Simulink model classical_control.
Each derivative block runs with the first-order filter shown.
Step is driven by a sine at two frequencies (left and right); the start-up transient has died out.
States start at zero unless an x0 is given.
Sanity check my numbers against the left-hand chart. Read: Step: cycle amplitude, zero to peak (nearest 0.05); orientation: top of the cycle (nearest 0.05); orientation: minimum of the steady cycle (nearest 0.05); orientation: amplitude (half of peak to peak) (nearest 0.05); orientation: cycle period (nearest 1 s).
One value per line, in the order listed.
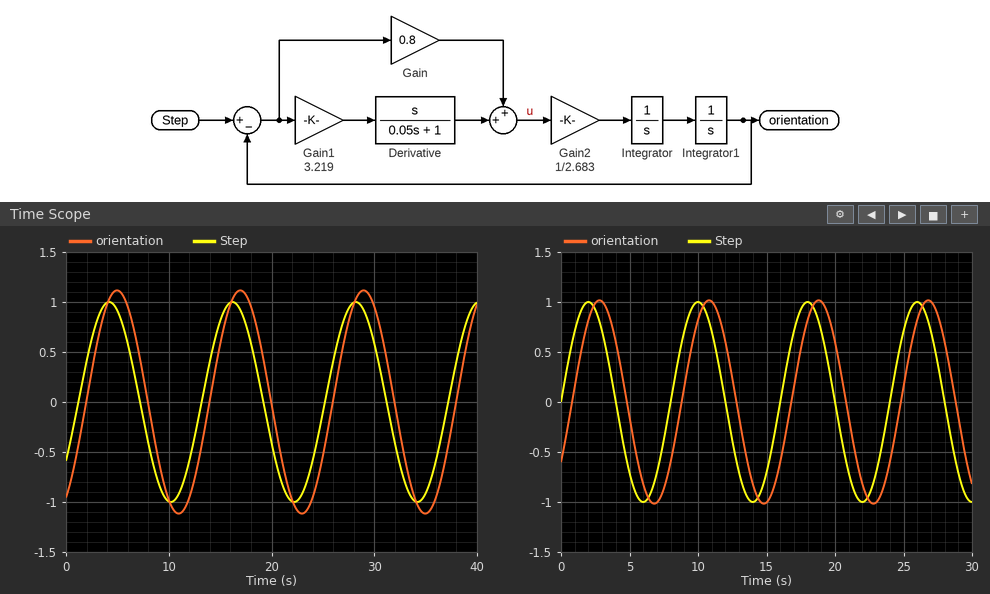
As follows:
1.00
1.10
-1.10
1.10
12 s
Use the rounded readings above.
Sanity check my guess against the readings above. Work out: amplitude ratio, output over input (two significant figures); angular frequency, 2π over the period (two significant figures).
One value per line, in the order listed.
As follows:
1.1
0.52 rad/s
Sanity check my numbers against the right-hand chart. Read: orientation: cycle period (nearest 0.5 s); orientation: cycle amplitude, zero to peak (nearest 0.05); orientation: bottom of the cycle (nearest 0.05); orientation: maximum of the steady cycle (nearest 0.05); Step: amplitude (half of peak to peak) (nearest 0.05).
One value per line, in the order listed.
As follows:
8.0 s
1.00
-1.00
1.00
1.00
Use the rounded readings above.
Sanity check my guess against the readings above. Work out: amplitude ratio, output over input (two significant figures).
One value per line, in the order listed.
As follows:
1.0
